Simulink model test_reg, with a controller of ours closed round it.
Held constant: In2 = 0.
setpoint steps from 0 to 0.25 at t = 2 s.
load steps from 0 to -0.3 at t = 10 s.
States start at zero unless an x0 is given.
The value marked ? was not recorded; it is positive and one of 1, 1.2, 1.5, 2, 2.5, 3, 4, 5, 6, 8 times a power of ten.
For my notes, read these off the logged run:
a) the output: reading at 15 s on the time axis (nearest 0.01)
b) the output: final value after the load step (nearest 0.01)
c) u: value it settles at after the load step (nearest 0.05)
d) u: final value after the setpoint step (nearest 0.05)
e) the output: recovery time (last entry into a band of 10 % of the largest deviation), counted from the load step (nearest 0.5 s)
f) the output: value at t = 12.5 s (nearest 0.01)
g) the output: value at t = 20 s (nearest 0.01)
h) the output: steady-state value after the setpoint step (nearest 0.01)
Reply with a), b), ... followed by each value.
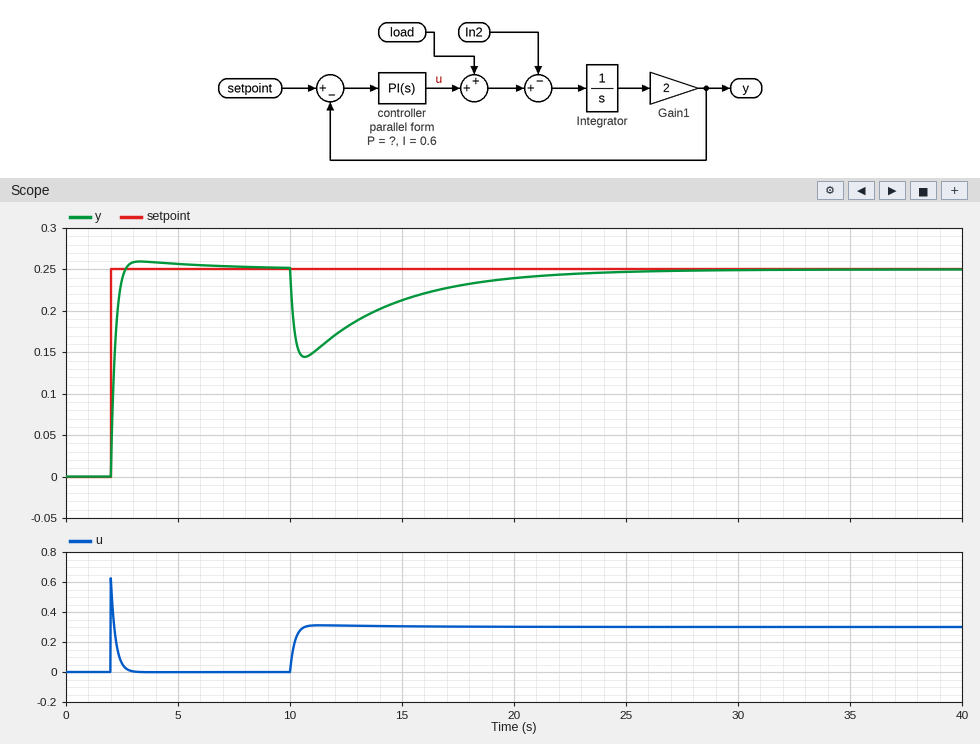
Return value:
a) 0.21
b) 0.25
c) 0.30
d) 0.00
e) 10.0 s
f) 0.18
g) 0.24
h) 0.25
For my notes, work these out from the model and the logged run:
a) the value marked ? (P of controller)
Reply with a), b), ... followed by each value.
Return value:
a) 2.5
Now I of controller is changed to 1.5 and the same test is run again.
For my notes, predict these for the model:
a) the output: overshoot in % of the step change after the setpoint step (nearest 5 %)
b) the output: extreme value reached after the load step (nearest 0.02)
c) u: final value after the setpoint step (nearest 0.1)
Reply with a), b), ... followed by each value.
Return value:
a) 10 %
b) 0.16
c) 0.0
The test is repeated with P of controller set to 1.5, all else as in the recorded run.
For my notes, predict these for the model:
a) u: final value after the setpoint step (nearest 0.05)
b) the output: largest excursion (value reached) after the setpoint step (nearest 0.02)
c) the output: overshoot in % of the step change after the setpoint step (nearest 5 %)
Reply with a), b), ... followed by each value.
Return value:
a) 0.00
b) 0.28
c) 10 %
